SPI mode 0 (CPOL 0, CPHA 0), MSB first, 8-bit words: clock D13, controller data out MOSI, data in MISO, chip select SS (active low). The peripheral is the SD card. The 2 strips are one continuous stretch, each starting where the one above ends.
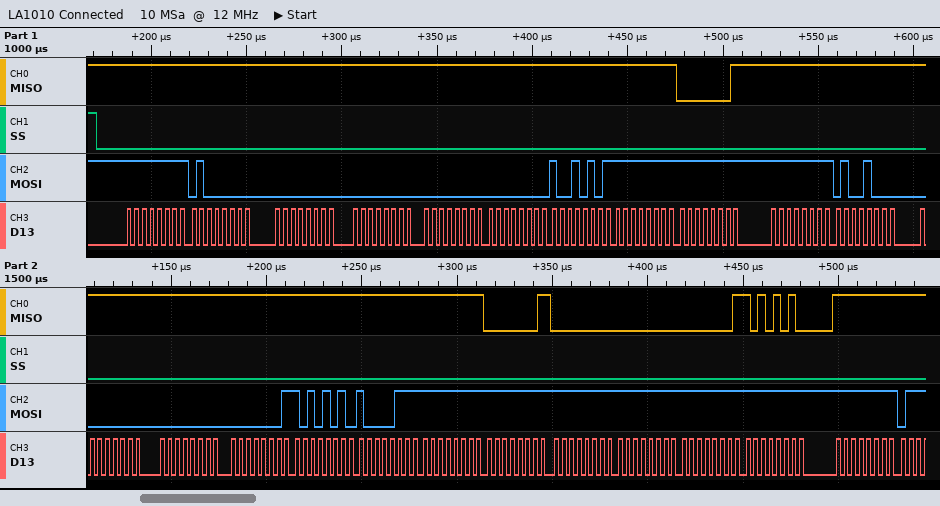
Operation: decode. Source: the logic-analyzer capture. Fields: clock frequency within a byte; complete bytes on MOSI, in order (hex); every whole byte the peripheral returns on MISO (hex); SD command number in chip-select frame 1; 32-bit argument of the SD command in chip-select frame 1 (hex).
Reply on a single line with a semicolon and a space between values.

250 kHz; FF 40 00 00 00 00 95 FF FF FF 48 00 00 01 AA 87 FF FF FF FF FF FF FF; FF FF FF FF FF FF FF FF 01 FF FF FF FF FF FF FF FF 01 00 00 01 AA FF; CMD0; 0x00000000
